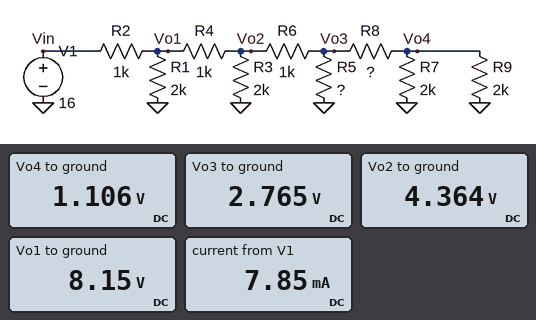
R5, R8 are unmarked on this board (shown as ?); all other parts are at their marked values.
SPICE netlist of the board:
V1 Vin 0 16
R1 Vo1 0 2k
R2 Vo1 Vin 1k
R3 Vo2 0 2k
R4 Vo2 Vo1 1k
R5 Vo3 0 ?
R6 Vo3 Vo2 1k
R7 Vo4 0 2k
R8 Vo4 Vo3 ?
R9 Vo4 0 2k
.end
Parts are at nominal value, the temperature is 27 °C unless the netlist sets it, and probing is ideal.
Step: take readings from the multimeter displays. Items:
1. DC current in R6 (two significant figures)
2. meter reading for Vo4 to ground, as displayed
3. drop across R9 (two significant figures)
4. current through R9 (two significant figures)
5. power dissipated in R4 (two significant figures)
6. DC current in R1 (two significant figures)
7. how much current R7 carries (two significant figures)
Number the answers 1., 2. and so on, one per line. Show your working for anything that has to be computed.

1. (4.364 V - 2.765 V) / 1 kΩ = 1.6 mA
2. 1.106 V
3. 1.106 V = 1.1 V
4. (1.106 V) / 2 kΩ = 550 µA
5. (8.15 V - 4.364 V)^2 / 1 kΩ = 14 mW
6. (8.15 V) / 2 kΩ = 4.1 mA
7. (1.106 V) / 2 kΩ = 550 µA
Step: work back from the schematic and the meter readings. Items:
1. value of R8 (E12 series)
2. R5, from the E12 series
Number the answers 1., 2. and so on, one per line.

1. 1.5 kΩ
2. 5.6 kΩ
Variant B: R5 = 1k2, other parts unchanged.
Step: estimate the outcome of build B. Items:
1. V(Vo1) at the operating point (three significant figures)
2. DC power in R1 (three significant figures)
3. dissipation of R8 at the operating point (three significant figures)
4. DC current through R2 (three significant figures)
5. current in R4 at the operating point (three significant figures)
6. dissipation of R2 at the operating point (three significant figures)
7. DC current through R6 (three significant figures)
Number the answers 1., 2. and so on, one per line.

1. 7.95 V
2. 31.6 mW
3. 722 µW
4. 8.05 mA
5. 4.08 mA
6. 64.8 mW
7. 2.14 mA
